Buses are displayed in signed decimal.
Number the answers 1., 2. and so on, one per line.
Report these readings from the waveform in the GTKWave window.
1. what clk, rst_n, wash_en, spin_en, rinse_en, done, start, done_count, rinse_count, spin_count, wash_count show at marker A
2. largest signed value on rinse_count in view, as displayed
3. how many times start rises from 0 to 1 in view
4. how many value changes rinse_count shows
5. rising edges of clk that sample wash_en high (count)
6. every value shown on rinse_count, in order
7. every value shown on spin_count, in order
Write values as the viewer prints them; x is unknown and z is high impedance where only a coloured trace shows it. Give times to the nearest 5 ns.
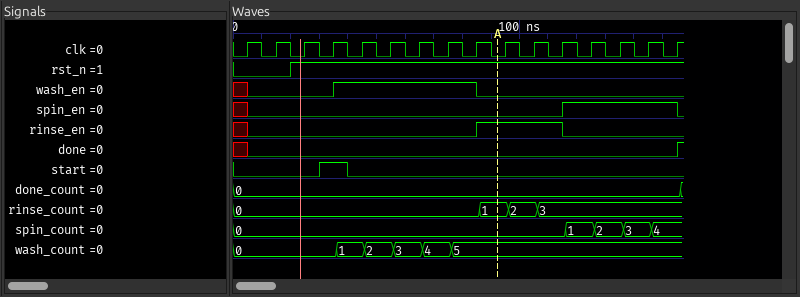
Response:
1. clk=0, rst_n=1, wash_en=0, spin_en=0, rinse_en=1, done=0, start=0, done_count=0, rinse_count=1, spin_count=0, wash_count=5
2. 3
3. 1
4. 3
5. 5
6. 0, 1, 2, 3
7. 0, 1, 2, 3, 4
